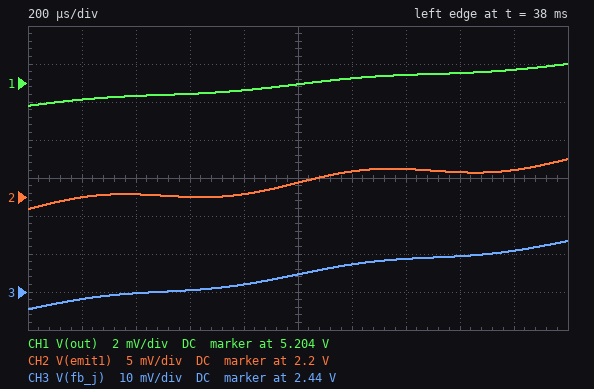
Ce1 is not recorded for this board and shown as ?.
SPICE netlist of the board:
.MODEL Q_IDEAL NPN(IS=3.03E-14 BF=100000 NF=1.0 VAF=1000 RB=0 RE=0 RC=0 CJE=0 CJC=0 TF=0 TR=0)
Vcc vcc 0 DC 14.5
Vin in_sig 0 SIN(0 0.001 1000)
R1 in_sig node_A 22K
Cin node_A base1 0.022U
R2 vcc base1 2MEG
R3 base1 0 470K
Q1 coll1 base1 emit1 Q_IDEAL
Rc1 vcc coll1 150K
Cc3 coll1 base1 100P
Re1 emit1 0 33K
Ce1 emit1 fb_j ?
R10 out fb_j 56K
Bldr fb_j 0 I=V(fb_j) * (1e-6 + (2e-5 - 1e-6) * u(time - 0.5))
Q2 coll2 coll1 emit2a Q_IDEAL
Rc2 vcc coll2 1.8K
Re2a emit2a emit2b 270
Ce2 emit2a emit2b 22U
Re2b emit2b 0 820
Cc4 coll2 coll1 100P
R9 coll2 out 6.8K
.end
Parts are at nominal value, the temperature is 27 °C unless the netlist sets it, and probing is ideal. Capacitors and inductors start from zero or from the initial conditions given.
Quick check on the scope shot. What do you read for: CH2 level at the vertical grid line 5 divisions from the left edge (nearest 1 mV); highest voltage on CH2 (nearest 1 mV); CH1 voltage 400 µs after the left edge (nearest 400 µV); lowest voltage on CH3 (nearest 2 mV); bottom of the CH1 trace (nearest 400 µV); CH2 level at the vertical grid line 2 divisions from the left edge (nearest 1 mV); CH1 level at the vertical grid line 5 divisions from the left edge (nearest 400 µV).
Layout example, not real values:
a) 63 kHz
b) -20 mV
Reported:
a) 2.202 V
b) 2.205 V
c) 5.2032 V
d) 2.436 V
e) 5.2028 V
f) 2.200 V
g) 5.2040 V
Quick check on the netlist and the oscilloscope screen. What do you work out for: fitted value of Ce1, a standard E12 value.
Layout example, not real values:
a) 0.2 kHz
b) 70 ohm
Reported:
a) 8.2 µF
